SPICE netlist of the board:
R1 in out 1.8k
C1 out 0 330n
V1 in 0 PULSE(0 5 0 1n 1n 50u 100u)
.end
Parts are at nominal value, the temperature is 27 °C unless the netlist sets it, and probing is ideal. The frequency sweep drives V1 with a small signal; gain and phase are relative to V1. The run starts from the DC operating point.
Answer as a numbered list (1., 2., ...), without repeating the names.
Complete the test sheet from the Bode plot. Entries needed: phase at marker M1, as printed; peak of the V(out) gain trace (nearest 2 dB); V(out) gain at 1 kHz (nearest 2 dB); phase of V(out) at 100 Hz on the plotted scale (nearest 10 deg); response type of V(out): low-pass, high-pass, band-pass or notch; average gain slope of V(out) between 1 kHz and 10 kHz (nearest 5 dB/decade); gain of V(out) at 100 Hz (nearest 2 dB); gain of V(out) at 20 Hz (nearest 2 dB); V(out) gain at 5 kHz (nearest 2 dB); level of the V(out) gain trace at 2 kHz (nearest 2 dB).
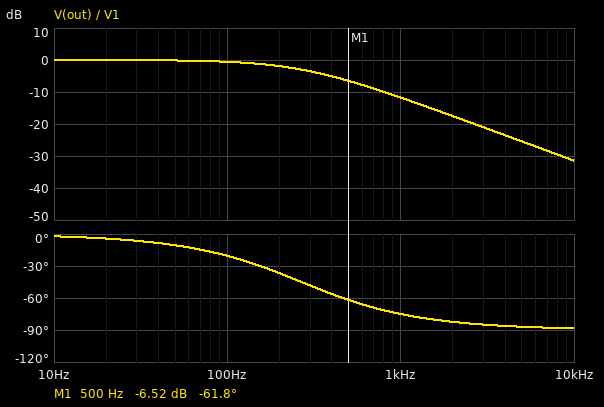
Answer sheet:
1. -61.8 deg
2. 0 dB
3. -12 dB
4. -20 deg
5. low-pass
6. -20 dB/decade
7. 0 dB
8. 0 dB
9. -26 dB
10. -18 dB
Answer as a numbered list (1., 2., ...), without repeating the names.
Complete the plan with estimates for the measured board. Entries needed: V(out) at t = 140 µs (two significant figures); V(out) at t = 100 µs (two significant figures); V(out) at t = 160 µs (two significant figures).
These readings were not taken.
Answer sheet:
1. 670 mV
2. 370 mV
3. 730 mV
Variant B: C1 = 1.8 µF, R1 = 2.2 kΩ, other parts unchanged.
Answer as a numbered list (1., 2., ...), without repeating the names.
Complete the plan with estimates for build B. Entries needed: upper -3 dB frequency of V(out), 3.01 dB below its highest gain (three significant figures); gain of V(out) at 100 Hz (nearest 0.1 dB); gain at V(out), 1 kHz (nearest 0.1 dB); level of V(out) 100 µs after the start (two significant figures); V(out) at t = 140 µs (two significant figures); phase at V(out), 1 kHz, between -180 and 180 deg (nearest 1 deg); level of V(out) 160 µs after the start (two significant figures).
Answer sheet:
1. 40.2 Hz
2. -8.6 dB
3. -27.9 dB
4. 62 mV
5. 110 mV
6. -88 deg
7. 120 mV
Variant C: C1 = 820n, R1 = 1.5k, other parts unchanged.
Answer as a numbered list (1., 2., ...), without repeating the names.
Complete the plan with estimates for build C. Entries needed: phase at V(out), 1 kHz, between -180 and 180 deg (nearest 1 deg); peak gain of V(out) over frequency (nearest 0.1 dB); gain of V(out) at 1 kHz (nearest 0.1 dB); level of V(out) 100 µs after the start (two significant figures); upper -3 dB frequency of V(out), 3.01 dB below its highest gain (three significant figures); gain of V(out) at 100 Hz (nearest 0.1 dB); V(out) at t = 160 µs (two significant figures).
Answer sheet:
1. -83 deg
2. 0 dB
3. -17.8 dB
4. 190 mV
5. 129 Hz
6. -2.0 dB
7. 380 mV
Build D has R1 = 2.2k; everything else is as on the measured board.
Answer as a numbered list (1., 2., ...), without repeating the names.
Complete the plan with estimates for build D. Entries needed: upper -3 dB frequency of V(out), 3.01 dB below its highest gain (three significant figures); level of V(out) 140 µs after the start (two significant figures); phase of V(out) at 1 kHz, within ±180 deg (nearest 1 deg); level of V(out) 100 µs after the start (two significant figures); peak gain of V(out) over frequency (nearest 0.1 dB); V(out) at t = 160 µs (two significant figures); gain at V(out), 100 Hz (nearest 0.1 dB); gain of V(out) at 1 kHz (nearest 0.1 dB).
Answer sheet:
1. 219 Hz
2. 560 mV
3. -78 deg
4. 310 mV
5. 0 dB
6. 610 mV
7. -0.8 dB
8. -13.4 dB
